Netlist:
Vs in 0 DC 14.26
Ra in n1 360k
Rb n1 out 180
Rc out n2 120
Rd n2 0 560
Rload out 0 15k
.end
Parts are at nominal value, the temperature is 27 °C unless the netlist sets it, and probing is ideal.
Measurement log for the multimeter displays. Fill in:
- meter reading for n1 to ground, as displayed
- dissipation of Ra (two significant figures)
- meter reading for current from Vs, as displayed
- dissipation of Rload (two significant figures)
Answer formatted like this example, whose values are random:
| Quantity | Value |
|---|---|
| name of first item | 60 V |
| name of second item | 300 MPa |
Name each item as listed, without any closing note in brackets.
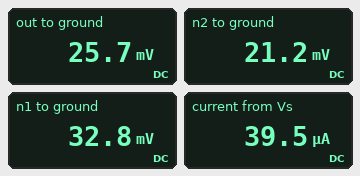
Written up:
| Quantity | Value |
|---|---|
| meter reading for n1 to ground, as displayed | 32.8 mV |
| dissipation of Ra | 560 µW |
| meter reading for current from Vs, as displayed | 39.5 µA |
| dissipation of Rload | 44 nW |
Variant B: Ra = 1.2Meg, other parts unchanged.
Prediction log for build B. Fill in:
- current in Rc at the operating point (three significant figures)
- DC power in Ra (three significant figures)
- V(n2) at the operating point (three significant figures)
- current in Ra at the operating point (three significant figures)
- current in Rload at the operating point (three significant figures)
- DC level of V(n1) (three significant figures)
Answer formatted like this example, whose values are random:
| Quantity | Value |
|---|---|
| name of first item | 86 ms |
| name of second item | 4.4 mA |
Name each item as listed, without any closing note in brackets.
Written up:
| Quantity | Value |
|---|---|
| current in Rc at the operating point | 11.4 µA |
| DC power in Ra | 169 µW |
| V(n2) at the operating point | 6.36 mV |
| current in Ra at the operating point | 11.9 µA |
| current in Rload at the operating point | 515 nA |
| DC level of V(n1) | 9.86 mV |
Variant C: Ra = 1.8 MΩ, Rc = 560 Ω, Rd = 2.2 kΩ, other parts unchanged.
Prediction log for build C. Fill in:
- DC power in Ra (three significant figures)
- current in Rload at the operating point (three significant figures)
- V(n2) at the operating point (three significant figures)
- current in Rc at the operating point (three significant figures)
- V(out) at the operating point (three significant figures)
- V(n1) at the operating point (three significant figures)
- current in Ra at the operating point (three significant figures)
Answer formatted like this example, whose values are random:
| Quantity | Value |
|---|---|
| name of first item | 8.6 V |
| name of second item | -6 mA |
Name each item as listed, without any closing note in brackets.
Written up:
| Quantity | Value |
|---|---|
| DC power in Ra | 113 µW |
| current in Rload at the operating point | 1.23 µA |
| V(n2) at the operating point | 14.7 mV |
| current in Rc at the operating point | 6.68 µA |
| V(out) at the operating point | 18.4 mV |
| V(n1) at the operating point | 19.9 mV |
| current in Ra at the operating point | 7.91 µA |
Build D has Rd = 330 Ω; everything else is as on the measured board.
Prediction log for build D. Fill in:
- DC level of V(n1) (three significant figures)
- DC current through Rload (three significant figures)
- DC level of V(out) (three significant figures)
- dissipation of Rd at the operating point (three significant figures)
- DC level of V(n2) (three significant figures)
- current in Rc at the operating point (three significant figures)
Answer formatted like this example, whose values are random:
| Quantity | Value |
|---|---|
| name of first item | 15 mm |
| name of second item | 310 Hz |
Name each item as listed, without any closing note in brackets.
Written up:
| Quantity | Value |
|---|---|
| DC level of V(n1) | 24.4 mV |
| DC current through Rload | 1.15 µA |
| DC level of V(out) | 17.3 mV |
| dissipation of Rd at the operating point | 486 nW |
| DC level of V(n2) | 12.7 mV |
| current in Rc at the operating point | 38.4 µA |
